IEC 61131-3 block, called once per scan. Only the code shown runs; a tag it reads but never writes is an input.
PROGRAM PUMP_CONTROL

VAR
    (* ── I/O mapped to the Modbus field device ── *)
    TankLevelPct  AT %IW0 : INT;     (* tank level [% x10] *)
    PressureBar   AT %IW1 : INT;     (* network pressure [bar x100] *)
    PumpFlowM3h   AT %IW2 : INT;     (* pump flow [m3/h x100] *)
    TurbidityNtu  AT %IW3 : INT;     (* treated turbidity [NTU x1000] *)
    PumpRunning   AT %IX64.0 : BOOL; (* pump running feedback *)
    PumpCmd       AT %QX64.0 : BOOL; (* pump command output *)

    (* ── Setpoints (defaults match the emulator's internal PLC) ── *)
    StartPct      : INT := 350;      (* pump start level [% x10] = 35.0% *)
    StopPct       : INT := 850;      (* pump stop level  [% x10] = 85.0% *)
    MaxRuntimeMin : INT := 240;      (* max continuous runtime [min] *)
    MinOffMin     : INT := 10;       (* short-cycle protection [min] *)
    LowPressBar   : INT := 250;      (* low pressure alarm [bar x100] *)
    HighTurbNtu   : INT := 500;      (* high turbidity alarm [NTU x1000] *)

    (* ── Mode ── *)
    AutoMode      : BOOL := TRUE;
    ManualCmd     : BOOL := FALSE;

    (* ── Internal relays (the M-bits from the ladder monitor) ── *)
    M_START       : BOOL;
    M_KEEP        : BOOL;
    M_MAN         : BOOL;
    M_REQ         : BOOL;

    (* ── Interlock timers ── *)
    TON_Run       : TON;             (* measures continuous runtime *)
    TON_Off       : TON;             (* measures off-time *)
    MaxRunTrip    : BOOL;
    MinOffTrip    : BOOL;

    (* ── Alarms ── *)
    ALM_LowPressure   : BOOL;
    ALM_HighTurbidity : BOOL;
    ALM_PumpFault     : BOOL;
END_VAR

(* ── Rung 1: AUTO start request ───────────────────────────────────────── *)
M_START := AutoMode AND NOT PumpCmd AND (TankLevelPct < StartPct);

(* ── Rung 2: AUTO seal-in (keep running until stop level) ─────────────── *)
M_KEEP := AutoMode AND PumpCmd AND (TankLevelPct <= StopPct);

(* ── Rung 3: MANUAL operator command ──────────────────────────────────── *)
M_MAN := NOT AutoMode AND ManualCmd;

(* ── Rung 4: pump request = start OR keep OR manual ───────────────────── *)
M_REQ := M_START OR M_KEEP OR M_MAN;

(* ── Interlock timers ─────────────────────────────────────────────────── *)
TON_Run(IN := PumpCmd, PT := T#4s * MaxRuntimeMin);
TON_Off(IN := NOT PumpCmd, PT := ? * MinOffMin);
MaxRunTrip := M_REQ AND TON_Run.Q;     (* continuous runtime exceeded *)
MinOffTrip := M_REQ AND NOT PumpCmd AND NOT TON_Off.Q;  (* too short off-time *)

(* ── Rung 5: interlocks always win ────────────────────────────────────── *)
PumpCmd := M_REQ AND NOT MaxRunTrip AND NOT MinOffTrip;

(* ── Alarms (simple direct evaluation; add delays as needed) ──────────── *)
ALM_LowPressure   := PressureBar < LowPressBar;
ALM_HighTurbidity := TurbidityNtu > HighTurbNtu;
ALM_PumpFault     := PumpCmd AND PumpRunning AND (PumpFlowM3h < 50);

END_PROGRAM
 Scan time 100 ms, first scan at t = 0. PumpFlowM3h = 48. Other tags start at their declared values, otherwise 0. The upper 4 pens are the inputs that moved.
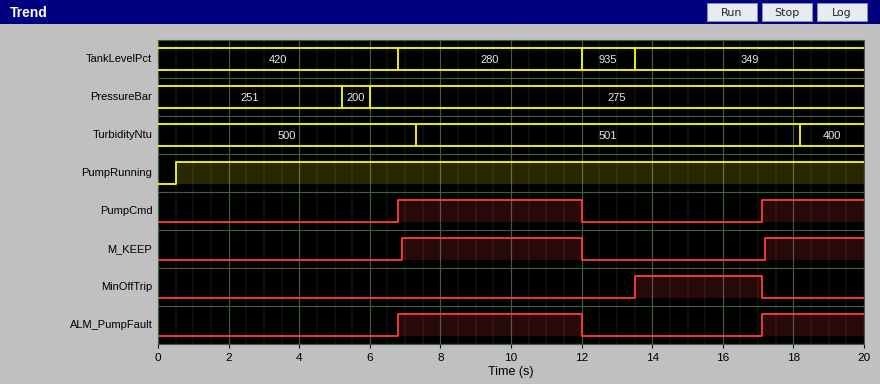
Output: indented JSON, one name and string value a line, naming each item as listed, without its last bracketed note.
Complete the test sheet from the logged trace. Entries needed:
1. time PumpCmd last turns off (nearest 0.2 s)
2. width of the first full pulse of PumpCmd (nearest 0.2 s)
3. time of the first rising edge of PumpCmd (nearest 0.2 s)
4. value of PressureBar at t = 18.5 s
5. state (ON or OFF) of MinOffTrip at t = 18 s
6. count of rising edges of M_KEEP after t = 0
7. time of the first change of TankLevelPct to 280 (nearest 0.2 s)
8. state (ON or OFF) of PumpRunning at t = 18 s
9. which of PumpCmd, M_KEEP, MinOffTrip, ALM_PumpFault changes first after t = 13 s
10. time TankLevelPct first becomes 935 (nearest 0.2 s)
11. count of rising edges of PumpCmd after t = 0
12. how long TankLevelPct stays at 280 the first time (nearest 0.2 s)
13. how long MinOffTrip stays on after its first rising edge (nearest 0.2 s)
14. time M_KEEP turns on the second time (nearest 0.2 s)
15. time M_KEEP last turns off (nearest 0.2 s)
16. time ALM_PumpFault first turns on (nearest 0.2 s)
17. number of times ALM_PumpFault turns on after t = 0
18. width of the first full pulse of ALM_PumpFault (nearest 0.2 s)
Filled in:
{
  "time PumpCmd last turns off": "12.0 s",
  "width of the first full pulse of PumpCmd": "5.2 s",
  "time of the first rising edge of PumpCmd": "6.8 s",
  "value of PressureBar at t = 18.5 s": "275",
  "state (ON or OFF) of MinOffTrip at t = 18 s": "OFF",
  "count of rising edges of M_KEEP after t = 0": "2",
  "time of the first change of TankLevelPct to 280": "6.8 s",
  "state (ON or OFF) of PumpRunning at t = 18 s": "ON",
  "which of PumpCmd, M_KEEP, MinOffTrip, ALM_PumpFault changes first after t = 13 s": "MinOffTrip",
  "time TankLevelPct first becomes 935": "12.0 s",
  "count of rising edges of PumpCmd after t = 0": "2",
  "how long TankLevelPct stays at 280 the first time": "5.2 s",
  "how long MinOffTrip stays on after its first rising edge": "3.6 s",
  "time M_KEEP turns on the second time": "17.2 s",
  "time M_KEEP last turns off": "12.0 s",
  "time ALM_PumpFault first turns on": "6.8 s",
  "number of times ALM_PumpFault turns on after t = 0": "2",
  "width of the first full pulse of ALM_PumpFault": "5.2 s"
}
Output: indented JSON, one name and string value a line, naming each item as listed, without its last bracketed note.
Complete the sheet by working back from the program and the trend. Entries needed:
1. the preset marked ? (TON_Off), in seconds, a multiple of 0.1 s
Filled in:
{
  "the preset marked ? (TON_Off), in seconds, a multiple of 0.1 s": "0.5 s"
}
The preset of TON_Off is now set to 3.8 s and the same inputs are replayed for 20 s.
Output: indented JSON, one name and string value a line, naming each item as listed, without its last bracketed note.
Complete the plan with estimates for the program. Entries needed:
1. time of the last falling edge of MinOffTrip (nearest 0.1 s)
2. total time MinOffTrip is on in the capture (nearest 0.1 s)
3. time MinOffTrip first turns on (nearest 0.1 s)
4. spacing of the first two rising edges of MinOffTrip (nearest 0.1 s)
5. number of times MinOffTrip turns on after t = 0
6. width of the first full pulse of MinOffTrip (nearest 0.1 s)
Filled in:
{
  "time of the last falling edge of MinOffTrip": "12.0 s",
  "total time MinOffTrip is on in the capture": "11.7 s",
  "time MinOffTrip first turns on": "6.8 s",
  "spacing of the first two rising edges of MinOffTrip": "6.7 s",
  "number of times MinOffTrip turns on after t = 0": "2",
  "width of the first full pulse of MinOffTrip": "5.2 s"
}
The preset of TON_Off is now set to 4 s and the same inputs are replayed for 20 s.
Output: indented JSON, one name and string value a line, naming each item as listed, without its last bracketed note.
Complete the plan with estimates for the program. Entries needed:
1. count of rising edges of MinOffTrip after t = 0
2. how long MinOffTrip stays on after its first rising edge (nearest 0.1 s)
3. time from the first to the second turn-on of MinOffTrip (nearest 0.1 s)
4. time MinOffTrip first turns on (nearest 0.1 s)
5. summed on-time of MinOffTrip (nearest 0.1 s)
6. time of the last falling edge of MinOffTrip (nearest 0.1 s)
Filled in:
{
  "count of rising edges of MinOffTrip after t = 0": "2",
  "how long MinOffTrip stays on after its first rising edge": "5.2 s",
  "time from the first to the second turn-on of MinOffTrip": "6.7 s",
  "time MinOffTrip first turns on": "6.8 s",
  "summed on-time of MinOffTrip": "11.7 s",
  "time of the last falling edge of MinOffTrip": "12.0 s"
}
